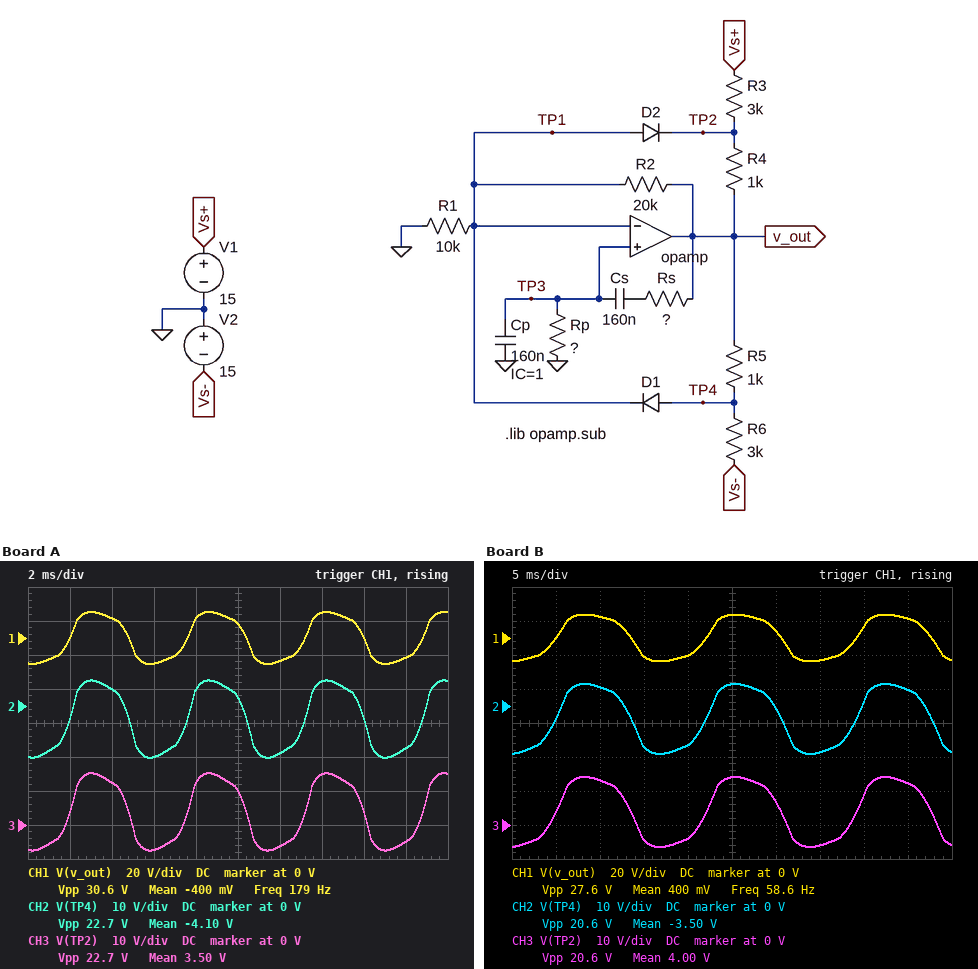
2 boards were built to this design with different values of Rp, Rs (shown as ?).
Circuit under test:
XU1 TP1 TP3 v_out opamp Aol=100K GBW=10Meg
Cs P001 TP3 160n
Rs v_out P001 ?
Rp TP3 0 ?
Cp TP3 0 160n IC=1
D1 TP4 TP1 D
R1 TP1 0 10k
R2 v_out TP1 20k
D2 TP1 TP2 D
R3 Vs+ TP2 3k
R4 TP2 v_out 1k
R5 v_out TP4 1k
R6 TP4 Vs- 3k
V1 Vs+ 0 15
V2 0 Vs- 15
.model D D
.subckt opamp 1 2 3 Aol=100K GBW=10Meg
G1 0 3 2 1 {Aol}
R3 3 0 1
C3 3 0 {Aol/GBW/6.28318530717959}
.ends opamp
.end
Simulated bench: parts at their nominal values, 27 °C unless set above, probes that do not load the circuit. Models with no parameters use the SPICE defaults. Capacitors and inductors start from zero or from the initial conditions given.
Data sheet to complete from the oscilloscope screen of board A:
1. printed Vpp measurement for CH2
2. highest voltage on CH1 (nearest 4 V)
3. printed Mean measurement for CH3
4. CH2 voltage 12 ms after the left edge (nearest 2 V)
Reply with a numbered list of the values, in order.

1. 22.7 V
2. 16 V
3. 3.50 V
4. -14 V
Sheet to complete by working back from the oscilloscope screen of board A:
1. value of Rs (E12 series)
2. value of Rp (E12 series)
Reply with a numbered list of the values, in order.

1. 3.3 kΩ
2. 8.2 kΩ
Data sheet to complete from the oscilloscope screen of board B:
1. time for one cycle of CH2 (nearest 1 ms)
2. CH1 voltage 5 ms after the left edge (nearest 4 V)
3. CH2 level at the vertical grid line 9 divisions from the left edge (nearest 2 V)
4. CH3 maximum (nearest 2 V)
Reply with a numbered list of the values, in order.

1. 17 ms
2. 0 V
3. 4 V
4. 14 V
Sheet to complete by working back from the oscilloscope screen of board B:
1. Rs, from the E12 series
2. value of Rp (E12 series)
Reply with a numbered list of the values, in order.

1. 12 kΩ
2. 22 kΩ
